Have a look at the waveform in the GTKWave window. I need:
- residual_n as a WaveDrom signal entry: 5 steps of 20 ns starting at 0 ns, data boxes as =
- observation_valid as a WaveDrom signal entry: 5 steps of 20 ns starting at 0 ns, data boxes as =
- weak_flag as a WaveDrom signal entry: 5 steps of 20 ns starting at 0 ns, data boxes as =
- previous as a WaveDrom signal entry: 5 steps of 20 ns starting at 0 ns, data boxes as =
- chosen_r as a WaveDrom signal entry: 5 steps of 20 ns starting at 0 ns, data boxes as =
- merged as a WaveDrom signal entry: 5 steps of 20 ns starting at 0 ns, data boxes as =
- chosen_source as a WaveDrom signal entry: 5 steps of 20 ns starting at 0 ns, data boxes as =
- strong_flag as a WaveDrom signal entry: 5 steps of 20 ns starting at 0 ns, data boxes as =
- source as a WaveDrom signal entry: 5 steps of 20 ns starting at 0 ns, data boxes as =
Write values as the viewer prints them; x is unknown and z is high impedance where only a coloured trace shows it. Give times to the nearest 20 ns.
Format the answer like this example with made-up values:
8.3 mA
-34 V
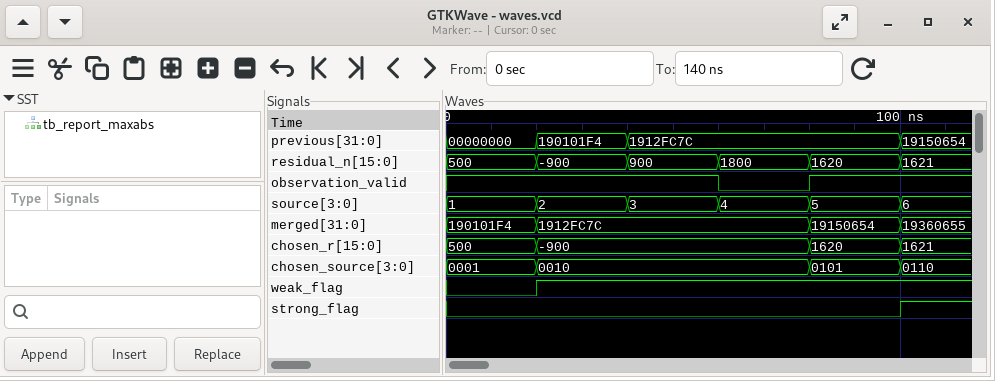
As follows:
{name: 'residual_n', wave: '=====', data: '500 -900 900 1800 1620'}
{name: 'observation_valid', wave: '1..01'}
{name: 'weak_flag', wave: '01...'}
{name: 'previous', wave: '===..', data: '00000000 190101F4 1912FC7C'}
{name: 'chosen_r', wave: '==..=', data: '500 -900 1620'}
{name: 'merged', wave: '==..=', data: '190101F4 1912FC7C 19150654'}
{name: 'chosen_source', wave: '==..=', data: '0001 0010 0101'}
{name: 'strong_flag', wave: '0....'}
{name: 'source', wave: '=====', data: '1 2 3 4 5'}
